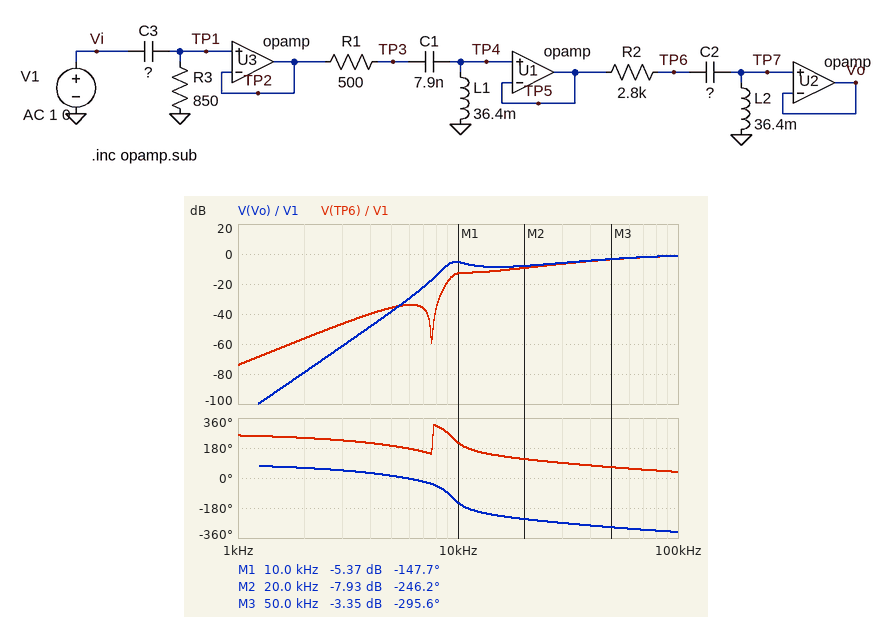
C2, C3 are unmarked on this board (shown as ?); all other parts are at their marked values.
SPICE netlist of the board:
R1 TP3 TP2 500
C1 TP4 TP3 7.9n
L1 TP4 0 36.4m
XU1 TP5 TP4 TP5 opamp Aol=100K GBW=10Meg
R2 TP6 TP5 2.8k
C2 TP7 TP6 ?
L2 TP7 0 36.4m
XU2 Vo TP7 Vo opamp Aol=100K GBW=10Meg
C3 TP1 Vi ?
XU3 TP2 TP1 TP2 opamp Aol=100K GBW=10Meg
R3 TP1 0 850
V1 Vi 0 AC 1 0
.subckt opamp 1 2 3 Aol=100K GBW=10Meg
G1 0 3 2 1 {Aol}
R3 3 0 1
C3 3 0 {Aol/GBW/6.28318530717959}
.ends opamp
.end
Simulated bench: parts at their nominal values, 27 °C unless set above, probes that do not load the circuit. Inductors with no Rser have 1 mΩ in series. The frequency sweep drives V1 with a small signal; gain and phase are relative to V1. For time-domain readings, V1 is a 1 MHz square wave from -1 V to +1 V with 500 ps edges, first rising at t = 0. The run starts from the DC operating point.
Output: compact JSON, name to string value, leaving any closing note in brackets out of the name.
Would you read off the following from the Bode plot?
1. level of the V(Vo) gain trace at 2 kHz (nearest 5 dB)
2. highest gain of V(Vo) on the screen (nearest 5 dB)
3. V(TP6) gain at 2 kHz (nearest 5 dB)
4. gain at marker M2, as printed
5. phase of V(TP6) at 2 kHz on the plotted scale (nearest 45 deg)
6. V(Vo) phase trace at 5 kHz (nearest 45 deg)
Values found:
{"level of the V(Vo) gain trace at 2 kHz": "-80 dB", "highest gain of V(Vo) on the screen": "0 dB", "V(TP6) gain at 2 kHz": "-55 dB", "gain at marker M2, as printed": "-7.93 dB", "phase of V(TP6) at 2 kHz on the plotted scale": "225 deg", "V(Vo) phase trace at 5 kHz": "0 deg"}
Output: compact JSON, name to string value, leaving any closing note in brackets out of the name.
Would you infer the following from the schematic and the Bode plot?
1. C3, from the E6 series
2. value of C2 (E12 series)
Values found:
{"C3, from the E6 series": "3.3 nF", "value of C2": "12 nF"}
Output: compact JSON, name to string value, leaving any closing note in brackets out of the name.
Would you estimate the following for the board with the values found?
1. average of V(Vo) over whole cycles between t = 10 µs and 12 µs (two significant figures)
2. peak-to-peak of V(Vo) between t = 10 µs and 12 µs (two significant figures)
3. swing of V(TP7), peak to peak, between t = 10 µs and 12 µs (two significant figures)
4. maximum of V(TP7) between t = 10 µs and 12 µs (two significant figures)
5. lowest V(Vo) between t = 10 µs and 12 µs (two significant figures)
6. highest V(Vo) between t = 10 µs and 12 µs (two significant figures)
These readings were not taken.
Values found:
{"average of V(Vo) over whole cycles between t = 10 µs and 12 µs": "-180 mV", "peak-to-peak of V(Vo) between t = 10 µs and 12 µs": "2.1 V", "swing of V(TP7), peak to peak, between t = 10 µs and 12 µs": "2.1 V", "maximum of V(TP7) between t = 10 µs and 12 µs": "880 mV", "lowest V(Vo) between t = 10 µs and 12 µs": "-1.2 V", "highest V(Vo) between t = 10 µs and 12 µs": "880 mV"}
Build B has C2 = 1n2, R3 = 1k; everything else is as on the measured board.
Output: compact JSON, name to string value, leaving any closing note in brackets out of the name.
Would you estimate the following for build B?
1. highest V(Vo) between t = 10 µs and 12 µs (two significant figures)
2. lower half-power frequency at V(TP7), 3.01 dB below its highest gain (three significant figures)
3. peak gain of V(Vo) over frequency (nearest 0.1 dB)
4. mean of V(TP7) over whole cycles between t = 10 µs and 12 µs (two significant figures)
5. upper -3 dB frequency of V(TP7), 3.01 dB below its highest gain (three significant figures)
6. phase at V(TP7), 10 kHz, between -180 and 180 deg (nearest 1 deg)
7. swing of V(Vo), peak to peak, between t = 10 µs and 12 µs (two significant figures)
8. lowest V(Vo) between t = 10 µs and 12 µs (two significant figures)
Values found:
{"highest V(Vo) between t = 10 µs and 12 µs": "710 mV", "lower half-power frequency at V(TP7), 3.01 dB below its highest gain": "21.4 kHz", "peak gain of V(Vo) over frequency": "0.9 dB", "mean of V(TP7) over whole cycles between t = 10 µs and 12 µs": "-340 mV", "upper -3 dB frequency of V(TP7), 3.01 dB below its highest gain": "5.21 MHz", "phase at V(TP7), 10 kHz, between -180 and 180 deg": "-55 deg", "swing of V(Vo), peak to peak, between t = 10 µs and 12 µs": "2.1 V", "lowest V(Vo) between t = 10 µs and 12 µs": "-1.4 V"}
